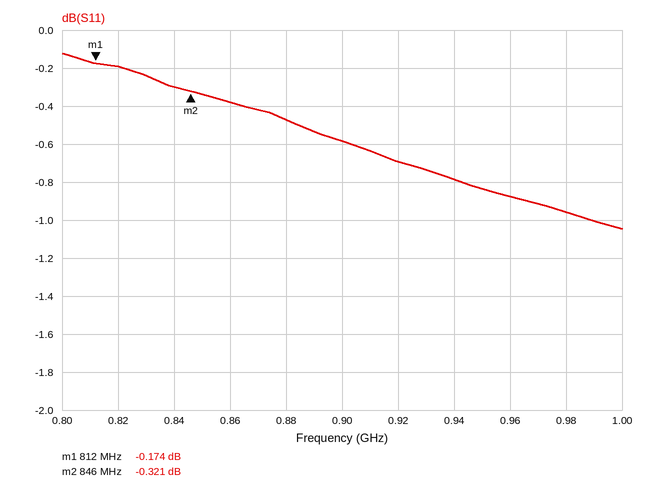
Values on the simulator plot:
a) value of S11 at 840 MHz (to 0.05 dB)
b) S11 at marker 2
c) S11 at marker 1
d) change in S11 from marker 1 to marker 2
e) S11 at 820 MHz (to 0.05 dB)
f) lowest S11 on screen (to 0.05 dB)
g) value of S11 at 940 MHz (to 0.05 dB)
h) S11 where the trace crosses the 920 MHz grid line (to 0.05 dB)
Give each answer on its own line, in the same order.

-0.30 dB
-0.321 dB
-0.174 dB
-0.147 dB
-0.20 dB
-1.05 dB
-0.80 dB
-0.70 dB
